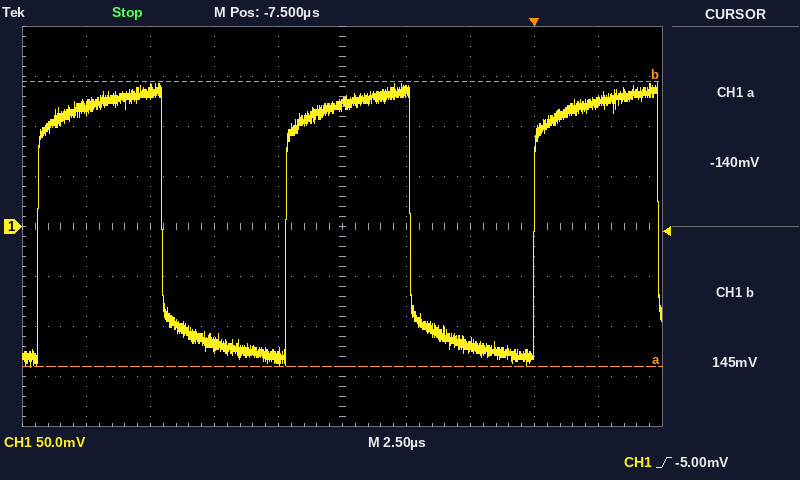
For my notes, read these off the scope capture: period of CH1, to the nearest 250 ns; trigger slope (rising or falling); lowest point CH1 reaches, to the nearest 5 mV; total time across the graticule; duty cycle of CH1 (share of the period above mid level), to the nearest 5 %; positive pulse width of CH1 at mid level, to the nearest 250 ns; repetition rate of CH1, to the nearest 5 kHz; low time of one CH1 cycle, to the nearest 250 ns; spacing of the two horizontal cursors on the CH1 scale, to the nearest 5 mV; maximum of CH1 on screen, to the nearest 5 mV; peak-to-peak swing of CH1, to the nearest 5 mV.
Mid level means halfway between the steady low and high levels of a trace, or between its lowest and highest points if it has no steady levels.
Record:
9.75 µs
rising
-140 mV
25 µs
50 %
4.75 µs
105 kHz
4.75 µs
285 mV
145 mV
285 mV
